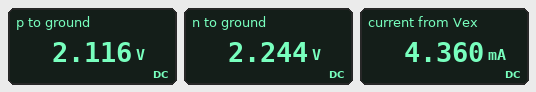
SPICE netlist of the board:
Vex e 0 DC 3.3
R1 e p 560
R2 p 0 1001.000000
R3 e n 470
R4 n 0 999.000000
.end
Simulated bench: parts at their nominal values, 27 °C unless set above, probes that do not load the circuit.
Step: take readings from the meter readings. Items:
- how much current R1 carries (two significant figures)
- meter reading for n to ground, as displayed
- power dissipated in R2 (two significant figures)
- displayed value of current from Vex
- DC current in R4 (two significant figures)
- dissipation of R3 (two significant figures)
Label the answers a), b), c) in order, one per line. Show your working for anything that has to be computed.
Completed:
a) (3.3 V - 2.116 V) / 560 Ω = 2.1 mA
b) 2.244 V
c) (2.116 V)^2 / 1.001 kΩ = 4.5 mW
d) 4.360 mA
e) (2.244 V) / 999 Ω = 2.2 mA
f) (3.3 V - 2.244 V)^2 / 470 Ω = 2.4 mW
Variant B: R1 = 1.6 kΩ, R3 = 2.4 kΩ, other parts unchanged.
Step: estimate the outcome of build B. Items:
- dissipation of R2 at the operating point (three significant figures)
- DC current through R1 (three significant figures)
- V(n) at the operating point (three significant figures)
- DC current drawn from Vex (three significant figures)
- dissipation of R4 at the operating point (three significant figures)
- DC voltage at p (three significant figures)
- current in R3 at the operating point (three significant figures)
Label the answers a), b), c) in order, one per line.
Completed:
a) 1.61 mW
b) 1.27 mA
c) 970 mV
d) 2.24 mA
e) 942 µW
f) 1.27 V
g) 971 µA
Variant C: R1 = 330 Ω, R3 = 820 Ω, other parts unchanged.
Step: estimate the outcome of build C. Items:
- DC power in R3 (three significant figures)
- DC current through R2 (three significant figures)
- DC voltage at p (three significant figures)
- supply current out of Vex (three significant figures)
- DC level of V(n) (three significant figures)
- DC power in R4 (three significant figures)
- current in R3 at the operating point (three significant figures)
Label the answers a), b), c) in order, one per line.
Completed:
a) 2.70 mW
b) 2.48 mA
c) 2.48 V
d) 4.29 mA
e) 1.81 V
f) 3.29 mW
g) 1.81 mA
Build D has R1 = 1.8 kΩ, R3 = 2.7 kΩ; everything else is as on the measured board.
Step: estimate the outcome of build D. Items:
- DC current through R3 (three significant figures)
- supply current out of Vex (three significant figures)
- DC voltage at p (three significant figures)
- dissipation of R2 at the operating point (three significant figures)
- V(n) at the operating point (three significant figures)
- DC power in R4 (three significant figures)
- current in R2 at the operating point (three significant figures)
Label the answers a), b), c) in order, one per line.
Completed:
a) 892 µA
b) 2.07 mA
c) 1.18 V
d) 1.39 mW
e) 891 mV
f) 795 µW
g) 1.18 mA
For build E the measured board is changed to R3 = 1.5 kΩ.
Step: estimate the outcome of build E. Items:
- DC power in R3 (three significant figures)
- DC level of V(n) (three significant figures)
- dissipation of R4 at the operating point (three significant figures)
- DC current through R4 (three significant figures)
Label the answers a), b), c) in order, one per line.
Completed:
a) 2.62 mW
b) 1.32 V
c) 1.74 mW
d) 1.32 mA
